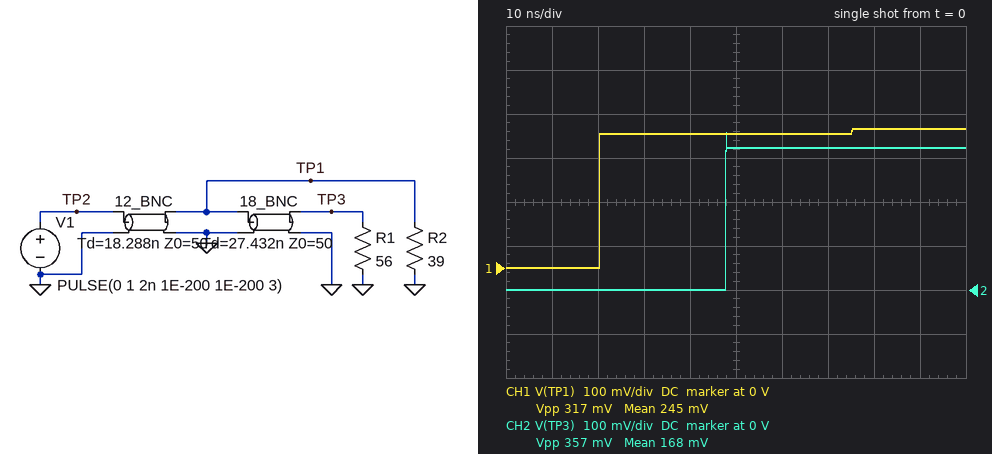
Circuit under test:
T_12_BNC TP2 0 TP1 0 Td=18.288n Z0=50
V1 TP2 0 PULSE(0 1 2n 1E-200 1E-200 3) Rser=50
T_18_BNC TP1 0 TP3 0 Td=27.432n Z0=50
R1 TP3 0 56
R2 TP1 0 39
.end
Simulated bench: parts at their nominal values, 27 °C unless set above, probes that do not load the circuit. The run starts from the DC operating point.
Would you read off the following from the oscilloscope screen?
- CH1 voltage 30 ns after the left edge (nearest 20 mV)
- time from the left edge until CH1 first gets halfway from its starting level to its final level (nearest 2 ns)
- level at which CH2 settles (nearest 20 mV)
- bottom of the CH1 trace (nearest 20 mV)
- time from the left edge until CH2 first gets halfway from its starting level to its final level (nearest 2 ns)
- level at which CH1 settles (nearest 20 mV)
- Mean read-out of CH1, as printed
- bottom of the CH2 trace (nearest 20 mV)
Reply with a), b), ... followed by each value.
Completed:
a) 300 mV
b) 20 ns
c) 320 mV
d) 0 V
e) 48 ns
f) 320 mV
g) 245 mV
h) 0 V
